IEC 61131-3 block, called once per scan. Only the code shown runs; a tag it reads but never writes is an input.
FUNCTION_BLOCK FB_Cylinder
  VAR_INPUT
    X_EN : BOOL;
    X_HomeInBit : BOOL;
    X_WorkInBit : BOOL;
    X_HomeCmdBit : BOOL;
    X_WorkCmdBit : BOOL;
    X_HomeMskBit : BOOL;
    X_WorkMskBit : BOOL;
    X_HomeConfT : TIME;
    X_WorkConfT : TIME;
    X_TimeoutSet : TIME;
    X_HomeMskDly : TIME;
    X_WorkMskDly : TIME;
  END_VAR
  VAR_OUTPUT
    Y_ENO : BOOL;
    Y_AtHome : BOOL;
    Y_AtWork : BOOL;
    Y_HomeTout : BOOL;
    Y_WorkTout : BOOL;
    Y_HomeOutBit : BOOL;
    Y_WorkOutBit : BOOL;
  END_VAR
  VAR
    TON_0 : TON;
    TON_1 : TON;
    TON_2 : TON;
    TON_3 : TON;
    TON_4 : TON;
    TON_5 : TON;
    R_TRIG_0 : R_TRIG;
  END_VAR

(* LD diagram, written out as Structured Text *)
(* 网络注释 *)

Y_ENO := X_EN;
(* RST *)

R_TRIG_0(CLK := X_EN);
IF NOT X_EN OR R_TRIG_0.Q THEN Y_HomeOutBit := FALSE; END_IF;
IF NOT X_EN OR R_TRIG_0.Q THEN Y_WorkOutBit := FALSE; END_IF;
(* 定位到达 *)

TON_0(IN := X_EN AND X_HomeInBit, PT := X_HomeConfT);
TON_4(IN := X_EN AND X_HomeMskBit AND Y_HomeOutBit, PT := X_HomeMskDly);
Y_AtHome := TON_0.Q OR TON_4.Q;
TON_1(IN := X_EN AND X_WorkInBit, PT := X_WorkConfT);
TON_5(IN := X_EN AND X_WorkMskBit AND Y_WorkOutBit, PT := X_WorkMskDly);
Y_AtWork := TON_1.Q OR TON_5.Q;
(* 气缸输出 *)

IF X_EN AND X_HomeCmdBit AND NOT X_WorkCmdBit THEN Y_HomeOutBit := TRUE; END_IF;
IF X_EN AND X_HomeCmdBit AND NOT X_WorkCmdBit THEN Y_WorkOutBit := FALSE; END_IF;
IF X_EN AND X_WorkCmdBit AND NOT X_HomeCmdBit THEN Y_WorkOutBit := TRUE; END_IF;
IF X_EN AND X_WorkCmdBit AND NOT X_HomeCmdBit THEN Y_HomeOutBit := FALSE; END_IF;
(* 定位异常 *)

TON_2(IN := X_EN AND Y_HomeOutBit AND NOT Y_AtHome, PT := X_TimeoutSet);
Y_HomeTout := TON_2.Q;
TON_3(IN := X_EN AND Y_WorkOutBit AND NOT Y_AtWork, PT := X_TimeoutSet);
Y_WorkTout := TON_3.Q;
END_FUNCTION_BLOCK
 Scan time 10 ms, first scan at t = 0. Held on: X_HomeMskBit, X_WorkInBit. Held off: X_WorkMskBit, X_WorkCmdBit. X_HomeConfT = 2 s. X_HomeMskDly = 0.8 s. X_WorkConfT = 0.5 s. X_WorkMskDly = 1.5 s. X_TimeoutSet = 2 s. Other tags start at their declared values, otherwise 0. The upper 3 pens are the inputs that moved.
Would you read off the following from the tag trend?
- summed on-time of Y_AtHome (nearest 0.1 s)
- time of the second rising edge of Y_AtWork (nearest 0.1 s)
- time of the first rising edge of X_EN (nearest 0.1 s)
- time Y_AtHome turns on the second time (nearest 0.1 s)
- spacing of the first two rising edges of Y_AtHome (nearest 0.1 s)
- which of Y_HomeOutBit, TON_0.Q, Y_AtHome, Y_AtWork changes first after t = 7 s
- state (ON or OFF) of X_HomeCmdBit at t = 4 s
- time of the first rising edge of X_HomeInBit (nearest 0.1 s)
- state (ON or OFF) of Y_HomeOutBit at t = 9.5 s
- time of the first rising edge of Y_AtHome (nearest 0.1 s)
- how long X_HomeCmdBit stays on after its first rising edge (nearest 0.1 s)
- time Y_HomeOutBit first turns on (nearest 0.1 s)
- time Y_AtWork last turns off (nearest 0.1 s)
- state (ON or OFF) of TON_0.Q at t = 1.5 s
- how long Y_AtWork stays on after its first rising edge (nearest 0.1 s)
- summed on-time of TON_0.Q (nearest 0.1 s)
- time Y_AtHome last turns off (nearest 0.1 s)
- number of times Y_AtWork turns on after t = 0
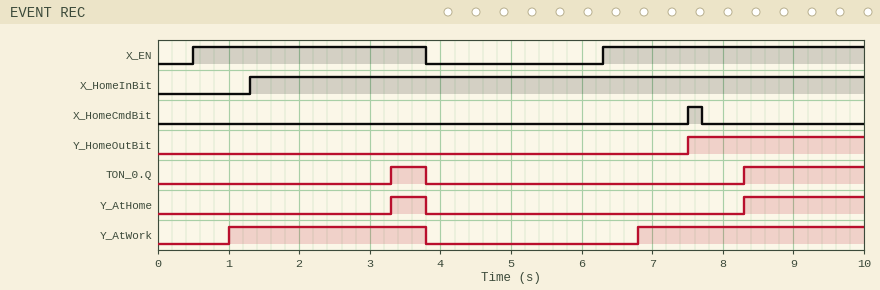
2.2 s
6.8 s
0.5 s
8.3 s
5.0 s
Y_HomeOutBit
OFF
1.3 s
ON
3.3 s
0.2 s
7.5 s
3.8 s
OFF
2.8 s
2.2 s
3.8 s
2
